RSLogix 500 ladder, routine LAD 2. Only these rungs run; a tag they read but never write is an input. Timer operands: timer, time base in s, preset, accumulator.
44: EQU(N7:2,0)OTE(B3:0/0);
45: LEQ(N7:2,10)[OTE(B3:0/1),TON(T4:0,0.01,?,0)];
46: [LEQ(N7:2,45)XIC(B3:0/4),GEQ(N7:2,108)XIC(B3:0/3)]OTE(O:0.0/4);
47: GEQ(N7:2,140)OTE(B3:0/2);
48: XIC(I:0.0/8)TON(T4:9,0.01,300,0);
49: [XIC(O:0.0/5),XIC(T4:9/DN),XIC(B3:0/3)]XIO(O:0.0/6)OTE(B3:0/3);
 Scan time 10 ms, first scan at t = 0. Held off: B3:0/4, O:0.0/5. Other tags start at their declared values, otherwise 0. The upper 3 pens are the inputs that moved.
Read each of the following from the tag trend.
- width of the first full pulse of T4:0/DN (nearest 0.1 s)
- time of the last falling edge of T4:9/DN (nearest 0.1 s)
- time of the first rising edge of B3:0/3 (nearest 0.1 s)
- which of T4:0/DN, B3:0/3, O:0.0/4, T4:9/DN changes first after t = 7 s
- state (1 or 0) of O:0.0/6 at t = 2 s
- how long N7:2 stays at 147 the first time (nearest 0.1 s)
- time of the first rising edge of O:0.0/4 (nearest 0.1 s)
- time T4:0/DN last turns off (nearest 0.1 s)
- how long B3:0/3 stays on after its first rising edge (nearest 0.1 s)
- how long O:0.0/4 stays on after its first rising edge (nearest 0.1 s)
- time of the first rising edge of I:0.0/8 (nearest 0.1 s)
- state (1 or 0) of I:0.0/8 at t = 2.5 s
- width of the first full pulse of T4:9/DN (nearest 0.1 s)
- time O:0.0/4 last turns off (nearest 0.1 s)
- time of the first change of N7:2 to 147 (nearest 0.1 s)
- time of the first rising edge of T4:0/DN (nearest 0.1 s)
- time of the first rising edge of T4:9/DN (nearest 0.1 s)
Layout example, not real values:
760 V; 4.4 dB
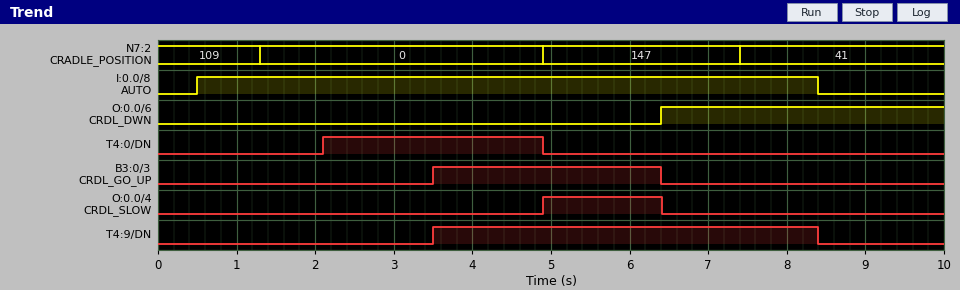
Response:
2.8 s; 8.4 s; 3.5 s; T4:9/DN; 0; 2.5 s; 4.9 s; 4.9 s; 2.9 s; 1.5 s; 0.5 s; 1; 4.9 s; 6.4 s; 4.9 s; 2.1 s; 3.5 s
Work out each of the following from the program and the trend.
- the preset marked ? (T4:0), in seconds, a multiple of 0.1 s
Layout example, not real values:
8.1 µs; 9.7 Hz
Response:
0.8 s
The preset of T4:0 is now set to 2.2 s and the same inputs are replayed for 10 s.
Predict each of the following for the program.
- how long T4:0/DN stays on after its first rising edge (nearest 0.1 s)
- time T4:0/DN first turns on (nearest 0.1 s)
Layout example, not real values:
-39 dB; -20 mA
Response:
1.4 s; 3.5 s
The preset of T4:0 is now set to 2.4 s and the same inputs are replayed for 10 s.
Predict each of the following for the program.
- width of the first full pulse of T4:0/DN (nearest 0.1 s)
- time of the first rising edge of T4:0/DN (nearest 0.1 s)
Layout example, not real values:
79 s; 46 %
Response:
1.2 s; 3.7 s
